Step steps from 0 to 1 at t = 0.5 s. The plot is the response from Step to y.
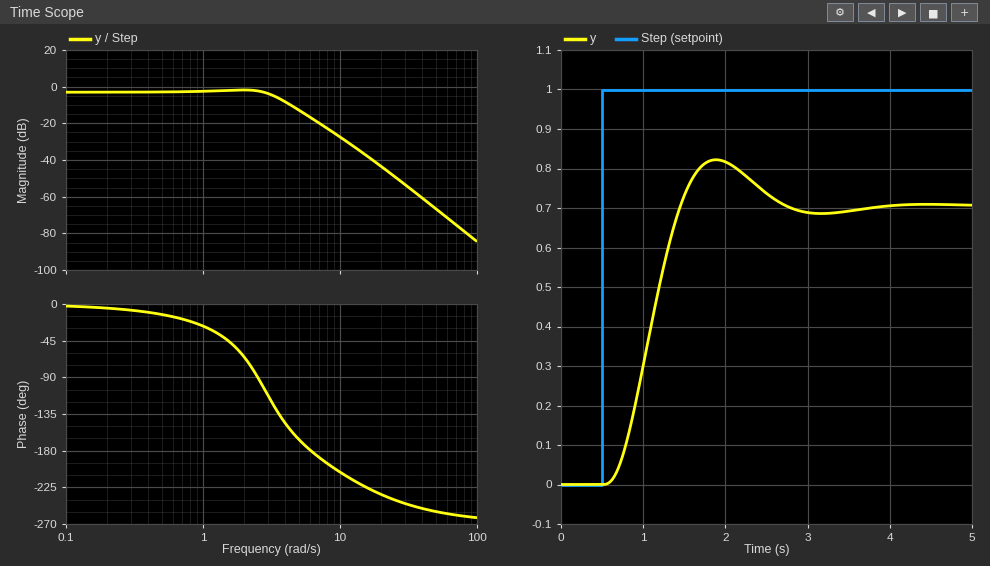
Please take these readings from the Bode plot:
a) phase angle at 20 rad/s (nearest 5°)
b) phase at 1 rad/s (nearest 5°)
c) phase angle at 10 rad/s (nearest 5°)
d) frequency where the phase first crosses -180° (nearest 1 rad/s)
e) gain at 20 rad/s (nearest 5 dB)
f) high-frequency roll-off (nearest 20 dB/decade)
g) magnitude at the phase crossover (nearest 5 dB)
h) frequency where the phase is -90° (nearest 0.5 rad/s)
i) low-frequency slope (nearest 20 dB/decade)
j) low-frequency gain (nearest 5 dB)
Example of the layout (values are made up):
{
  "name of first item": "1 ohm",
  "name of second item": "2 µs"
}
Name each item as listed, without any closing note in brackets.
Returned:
{
  "phase angle at 20 rad/s": "-235°",
  "phase at 1 rad/s": "-25°",
  "phase angle at 10 rad/s": "-205°",
  "frequency where the phase first crosses -180°": "6 rad/s",
  "gain at 20 rad/s": "-45 dB",
  "high-frequency roll-off": "-60 dB/decade",
  "magnitude at the phase crossover": "-15 dB",
  "frequency where the phase is -90°": "2.5 rad/s",
  "low-frequency slope": "0 dB/decade",
  "low-frequency gain": "-5 dB"
}
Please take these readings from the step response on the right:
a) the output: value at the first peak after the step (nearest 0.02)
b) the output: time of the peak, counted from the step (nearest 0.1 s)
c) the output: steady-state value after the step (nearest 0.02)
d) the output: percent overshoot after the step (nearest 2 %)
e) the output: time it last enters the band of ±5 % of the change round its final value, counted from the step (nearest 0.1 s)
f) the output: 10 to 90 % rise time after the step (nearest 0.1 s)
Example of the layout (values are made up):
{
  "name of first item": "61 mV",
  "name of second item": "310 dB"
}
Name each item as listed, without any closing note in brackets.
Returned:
{
  "the output: value at the first peak after the step": "0.82",
  "the output: time of the peak, counted from the step": "1.4 s",
  "the output: steady-state value after the step": "0.70",
  "the output: percent overshoot after the step": "16 %",
  "the output: time it last enters the band of ±5 % of the change round its final value, counted from the step": "2.0 s",
  "the output: 10 to 90 % rise time after the step": "0.6 s"
}
